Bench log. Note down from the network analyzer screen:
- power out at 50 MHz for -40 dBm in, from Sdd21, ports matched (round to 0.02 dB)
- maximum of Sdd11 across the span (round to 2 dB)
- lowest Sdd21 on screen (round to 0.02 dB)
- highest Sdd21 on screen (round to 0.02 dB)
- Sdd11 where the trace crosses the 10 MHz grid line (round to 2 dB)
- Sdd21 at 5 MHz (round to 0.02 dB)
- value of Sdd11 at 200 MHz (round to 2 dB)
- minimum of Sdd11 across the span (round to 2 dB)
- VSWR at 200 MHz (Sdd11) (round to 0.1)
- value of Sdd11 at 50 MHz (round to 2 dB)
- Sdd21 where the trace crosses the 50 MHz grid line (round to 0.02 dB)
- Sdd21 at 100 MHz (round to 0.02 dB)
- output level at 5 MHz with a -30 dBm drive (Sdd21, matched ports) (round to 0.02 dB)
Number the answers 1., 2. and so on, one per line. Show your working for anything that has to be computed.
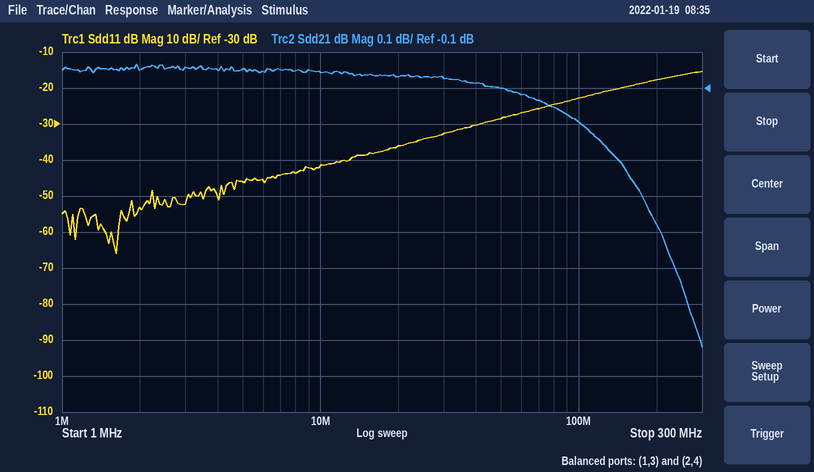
1. -40 dBm + (-0.10 dB) = -40.10 dBm
2. -16 dB
3. -0.82 dB
4. -0.04 dB
5. -42 dB
6. -0.04 dB
7. -18 dB
8. -66 dB
9. |Γ| = 10^(-18/20) = 0.1259; VSWR = (1 + 0.1259)/(1 − 0.1259) ≈ 1.3
10. -28 dB
11. -0.10 dB
12. -0.20 dB
13. -30 dBm + (-0.04 dB) = -30.04 dBm
